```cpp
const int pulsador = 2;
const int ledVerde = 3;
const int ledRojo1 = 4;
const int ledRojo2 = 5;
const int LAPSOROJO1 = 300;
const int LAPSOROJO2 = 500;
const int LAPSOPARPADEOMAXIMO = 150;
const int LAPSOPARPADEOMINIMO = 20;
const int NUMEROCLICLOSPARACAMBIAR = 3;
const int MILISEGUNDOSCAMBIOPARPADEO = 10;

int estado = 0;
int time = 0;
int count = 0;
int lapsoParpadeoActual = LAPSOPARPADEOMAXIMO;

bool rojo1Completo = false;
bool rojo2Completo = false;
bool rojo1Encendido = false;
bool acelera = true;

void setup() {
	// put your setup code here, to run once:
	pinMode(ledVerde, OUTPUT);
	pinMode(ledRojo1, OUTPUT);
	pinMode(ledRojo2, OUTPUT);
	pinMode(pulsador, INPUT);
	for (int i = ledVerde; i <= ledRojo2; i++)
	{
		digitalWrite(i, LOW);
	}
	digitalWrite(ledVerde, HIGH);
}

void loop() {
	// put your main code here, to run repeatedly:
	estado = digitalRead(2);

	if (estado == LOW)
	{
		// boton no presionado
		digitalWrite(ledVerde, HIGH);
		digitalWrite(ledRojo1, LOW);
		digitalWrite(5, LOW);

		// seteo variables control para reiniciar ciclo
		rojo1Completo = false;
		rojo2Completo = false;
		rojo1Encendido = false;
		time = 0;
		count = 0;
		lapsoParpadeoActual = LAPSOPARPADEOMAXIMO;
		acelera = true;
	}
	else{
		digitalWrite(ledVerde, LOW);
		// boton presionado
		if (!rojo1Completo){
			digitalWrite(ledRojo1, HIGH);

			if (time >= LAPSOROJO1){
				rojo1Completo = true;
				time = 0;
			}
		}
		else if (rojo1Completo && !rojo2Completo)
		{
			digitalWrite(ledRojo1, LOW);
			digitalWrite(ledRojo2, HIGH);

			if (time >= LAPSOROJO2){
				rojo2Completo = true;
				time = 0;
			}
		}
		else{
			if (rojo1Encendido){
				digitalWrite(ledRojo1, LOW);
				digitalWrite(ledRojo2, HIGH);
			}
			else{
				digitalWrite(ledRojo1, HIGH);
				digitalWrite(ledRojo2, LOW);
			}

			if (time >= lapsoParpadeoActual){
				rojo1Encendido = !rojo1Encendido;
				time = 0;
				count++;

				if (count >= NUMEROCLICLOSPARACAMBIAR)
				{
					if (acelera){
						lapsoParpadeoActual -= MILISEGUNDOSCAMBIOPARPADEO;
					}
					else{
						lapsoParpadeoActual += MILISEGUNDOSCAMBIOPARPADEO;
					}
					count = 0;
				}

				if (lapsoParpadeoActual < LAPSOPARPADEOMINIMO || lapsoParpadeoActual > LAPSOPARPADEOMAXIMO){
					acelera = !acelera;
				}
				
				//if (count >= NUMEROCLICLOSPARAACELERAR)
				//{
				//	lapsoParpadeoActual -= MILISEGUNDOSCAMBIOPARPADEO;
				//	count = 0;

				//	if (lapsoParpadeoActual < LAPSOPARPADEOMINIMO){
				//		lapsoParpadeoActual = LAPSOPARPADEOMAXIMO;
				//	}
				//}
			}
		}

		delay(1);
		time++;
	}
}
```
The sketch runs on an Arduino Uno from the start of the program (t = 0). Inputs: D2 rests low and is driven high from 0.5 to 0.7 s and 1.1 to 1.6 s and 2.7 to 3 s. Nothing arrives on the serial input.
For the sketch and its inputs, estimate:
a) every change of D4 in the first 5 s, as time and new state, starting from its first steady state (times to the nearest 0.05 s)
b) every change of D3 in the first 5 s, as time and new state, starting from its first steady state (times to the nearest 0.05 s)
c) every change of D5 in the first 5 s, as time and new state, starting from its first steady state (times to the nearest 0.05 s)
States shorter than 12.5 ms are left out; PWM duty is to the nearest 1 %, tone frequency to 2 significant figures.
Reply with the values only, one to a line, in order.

0 s low; 0.5 s high; 0.7 s low; 1.1 s high; 1.4 s low; 2.7 s high; 3 s low
0 s high; 0.5 s low; 0.7 s high; 1.1 s low; 1.6 s high; 2.7 s low; 3 s high
0 s low; 1.4 s high; 1.6 s low
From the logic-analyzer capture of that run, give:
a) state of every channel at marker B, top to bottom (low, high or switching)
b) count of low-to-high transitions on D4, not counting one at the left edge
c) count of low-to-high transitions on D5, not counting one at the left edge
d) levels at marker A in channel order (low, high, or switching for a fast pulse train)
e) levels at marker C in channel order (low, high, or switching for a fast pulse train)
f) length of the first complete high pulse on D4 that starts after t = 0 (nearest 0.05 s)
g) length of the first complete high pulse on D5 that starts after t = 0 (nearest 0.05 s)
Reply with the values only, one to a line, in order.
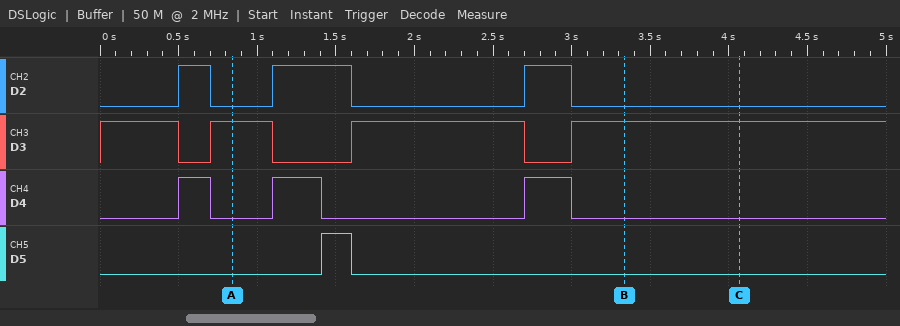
D2 low, D3 high, D4 low, D5 low
3
1
D2 low, D3 high, D4 low, D5 low
D2 low, D3 high, D4 low, D5 low
0.20 s
0.20 s
